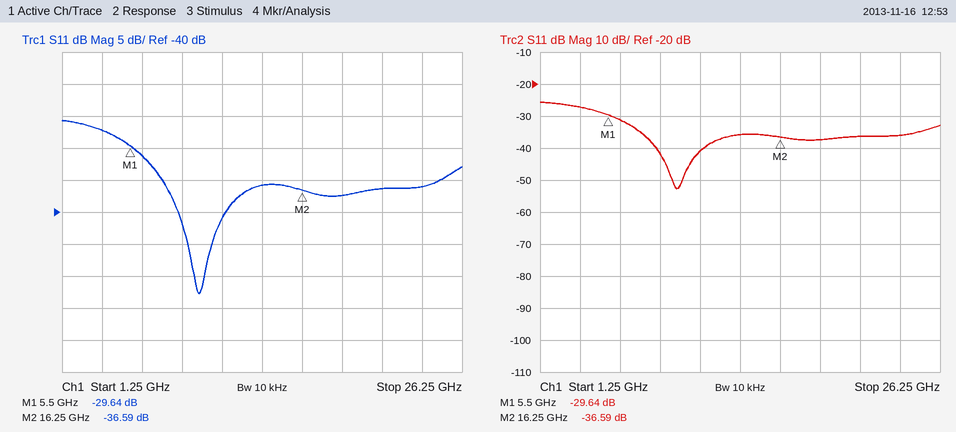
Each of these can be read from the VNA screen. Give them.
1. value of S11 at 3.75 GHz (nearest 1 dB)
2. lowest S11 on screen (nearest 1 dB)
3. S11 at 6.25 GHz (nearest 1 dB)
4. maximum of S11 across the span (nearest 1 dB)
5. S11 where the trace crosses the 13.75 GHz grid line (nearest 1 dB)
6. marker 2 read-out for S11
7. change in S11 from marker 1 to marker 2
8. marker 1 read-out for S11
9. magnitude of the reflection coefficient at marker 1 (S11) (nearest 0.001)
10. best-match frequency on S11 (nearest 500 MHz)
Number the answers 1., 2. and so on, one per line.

1. -27 dB
2. -53 dB
3. -31 dB
4. -26 dB
5. -36 dB
6. -36.59 dB
7. -6.95 dB
8. -29.64 dB
9. 0.033
10. 10.0 GHz
